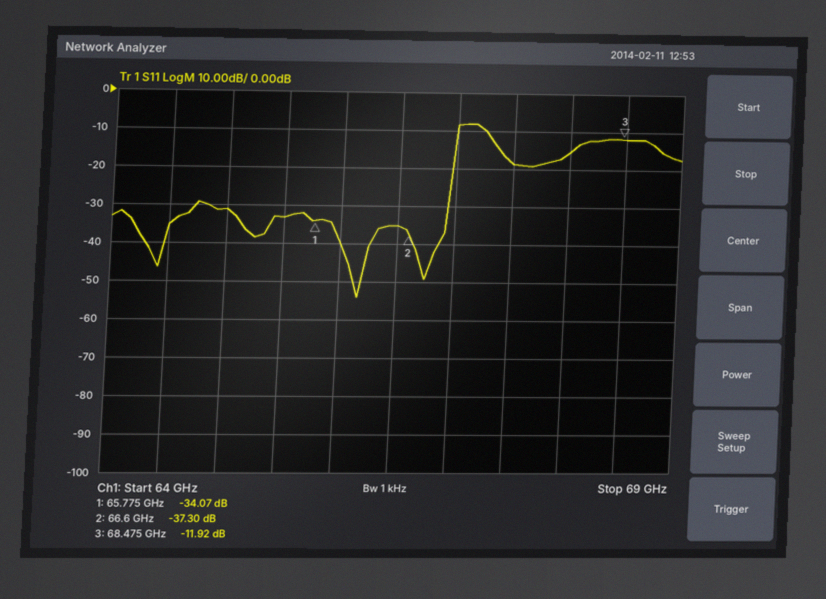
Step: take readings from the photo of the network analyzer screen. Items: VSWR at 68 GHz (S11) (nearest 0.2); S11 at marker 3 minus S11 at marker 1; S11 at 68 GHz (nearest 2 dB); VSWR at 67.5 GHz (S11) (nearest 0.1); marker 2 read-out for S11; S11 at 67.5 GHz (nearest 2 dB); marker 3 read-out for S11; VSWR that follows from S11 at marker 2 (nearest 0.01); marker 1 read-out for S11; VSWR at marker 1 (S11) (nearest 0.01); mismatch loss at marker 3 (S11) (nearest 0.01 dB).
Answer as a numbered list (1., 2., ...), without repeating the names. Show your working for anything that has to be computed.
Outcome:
1. |Γ| = 10^(-16/20) = 0.1585; VSWR = (1 + 0.1585)/(1 − 0.1585) ≈ 1.4
2. -11.92 − (-34.07) = 22.15 dB
3. -16 dB
4. |Γ| = 10^(-18/20) = 0.1259; VSWR = (1 + 0.1259)/(1 − 0.1259) ≈ 1.3
5. -37.30 dB
6. -18 dB
7. -11.92 dB
8. (1 + 0.0136)/(1 − 0.0136) ≈ 1.03
9. -34.07 dB
10. (1 + 0.0198)/(1 − 0.0198) ≈ 1.04
11. −10 log10(1 − 10^(-11.92/10)) ≈ 0.29 dB
